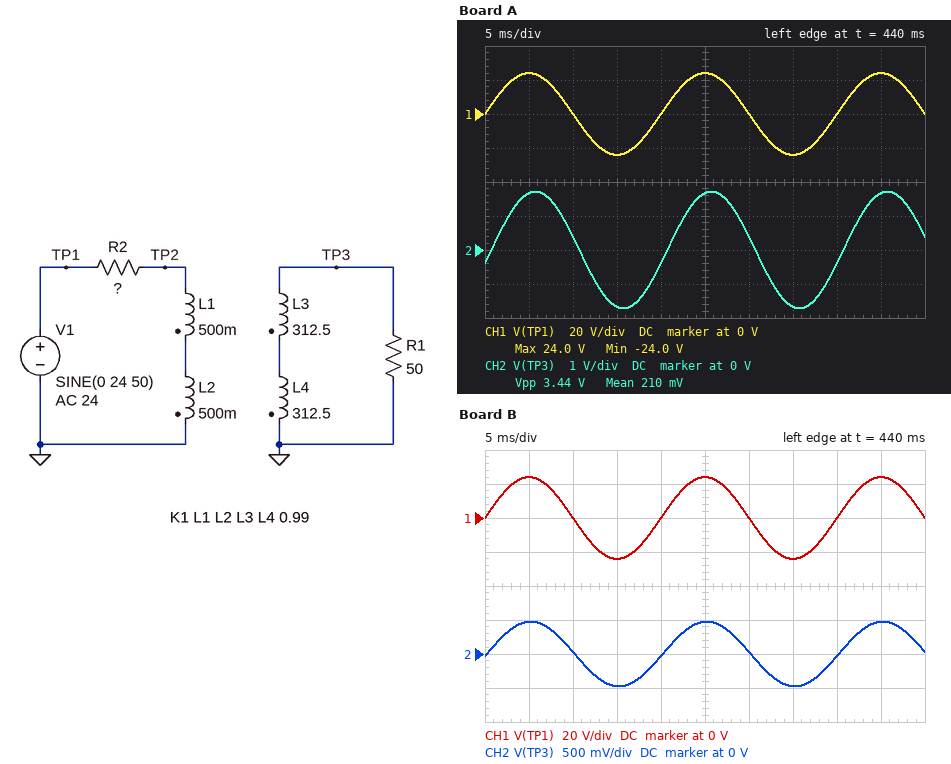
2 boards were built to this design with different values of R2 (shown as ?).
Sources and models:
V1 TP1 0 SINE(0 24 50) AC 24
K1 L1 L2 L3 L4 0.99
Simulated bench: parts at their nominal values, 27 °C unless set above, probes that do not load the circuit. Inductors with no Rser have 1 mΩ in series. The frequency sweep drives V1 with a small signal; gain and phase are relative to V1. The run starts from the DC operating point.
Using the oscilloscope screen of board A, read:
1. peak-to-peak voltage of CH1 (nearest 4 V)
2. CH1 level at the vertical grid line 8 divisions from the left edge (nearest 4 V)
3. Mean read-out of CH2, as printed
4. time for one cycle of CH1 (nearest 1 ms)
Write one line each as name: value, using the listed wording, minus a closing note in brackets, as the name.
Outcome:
peak-to-peak voltage of CH1: 48 V
CH1 level at the vertical grid line 8 divisions from the left edge: 0 V
Mean read-out of CH2, as printed: 210 mV
time for one cycle of CH1: 20 ms
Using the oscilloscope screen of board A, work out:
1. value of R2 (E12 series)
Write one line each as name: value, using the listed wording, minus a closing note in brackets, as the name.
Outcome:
value of R2: 27 Ω
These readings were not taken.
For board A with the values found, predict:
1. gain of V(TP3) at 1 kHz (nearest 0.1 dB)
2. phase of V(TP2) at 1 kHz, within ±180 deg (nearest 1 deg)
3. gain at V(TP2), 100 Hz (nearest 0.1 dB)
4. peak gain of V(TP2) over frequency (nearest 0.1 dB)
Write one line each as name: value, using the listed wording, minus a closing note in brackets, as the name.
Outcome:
gain of V(TP3) at 1 kHz: -36.2 dB
phase of V(TP2) at 1 kHz, within ±180 deg: 12 deg
gain at V(TP2), 100 Hz: -7.5 dB
peak gain of V(TP2) over frequency: 0 dB
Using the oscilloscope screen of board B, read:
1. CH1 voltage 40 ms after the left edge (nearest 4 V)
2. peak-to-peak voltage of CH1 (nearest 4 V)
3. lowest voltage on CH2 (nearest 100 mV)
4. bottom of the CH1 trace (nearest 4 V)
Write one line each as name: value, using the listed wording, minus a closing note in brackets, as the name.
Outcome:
CH1 voltage 40 ms after the left edge: 0 V
peak-to-peak voltage of CH1: 48 V
lowest voltage on CH2: -500 mV
bottom of the CH1 trace: -24 V
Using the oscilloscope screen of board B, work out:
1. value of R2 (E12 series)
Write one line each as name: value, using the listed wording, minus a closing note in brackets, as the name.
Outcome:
value of R2: 100 Ω
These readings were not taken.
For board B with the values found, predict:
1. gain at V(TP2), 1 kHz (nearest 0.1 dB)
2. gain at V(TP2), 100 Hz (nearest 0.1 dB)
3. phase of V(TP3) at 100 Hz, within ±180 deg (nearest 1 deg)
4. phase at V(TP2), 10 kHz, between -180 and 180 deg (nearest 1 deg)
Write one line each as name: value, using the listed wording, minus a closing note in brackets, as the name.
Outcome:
gain at V(TP2), 1 kHz: -2.1 dB
gain at V(TP2), 100 Hz: -18.1 dB
phase of V(TP3) at 100 Hz, within ±180 deg: -7 deg
phase at V(TP2), 10 kHz, between -180 and 180 deg: 5 deg
